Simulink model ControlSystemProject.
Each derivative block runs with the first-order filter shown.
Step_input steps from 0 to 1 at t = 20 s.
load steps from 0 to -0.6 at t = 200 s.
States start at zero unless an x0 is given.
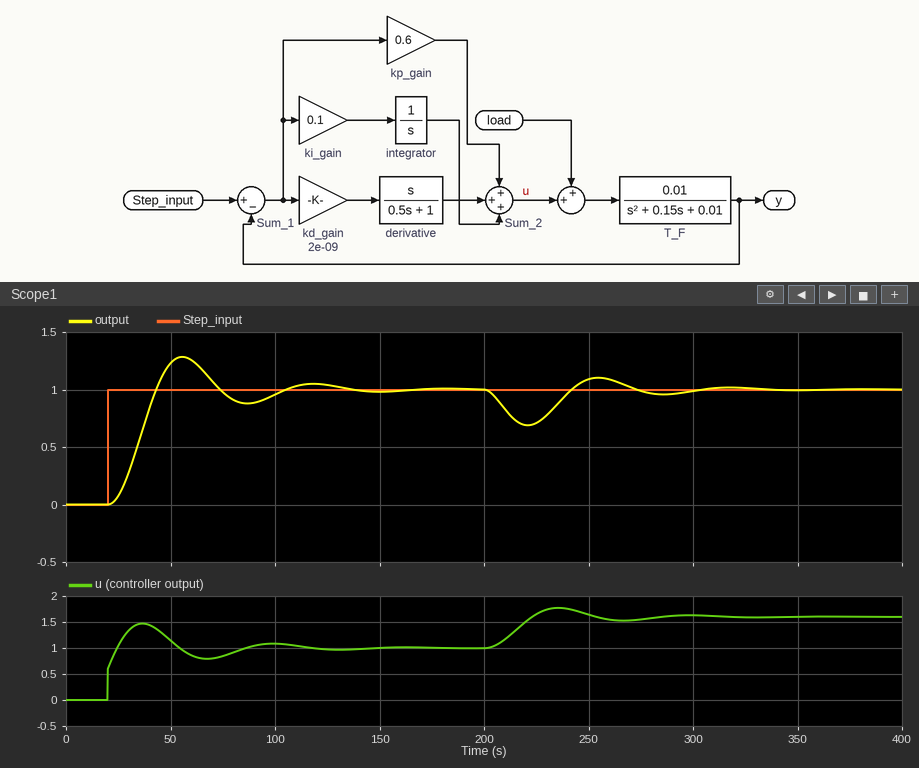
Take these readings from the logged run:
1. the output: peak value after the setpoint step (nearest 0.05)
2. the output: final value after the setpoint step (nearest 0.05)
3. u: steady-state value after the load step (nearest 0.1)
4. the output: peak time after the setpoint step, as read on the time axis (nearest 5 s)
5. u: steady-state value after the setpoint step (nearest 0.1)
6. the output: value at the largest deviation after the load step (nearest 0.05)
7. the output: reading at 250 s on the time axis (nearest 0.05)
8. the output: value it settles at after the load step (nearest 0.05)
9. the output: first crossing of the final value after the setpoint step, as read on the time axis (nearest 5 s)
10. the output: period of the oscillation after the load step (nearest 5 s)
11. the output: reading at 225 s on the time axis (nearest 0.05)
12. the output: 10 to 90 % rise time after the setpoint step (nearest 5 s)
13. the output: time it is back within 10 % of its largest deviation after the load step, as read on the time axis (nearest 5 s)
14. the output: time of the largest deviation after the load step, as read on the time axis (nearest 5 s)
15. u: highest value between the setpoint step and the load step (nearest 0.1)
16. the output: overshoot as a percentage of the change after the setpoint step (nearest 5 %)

1.30
1.00
1.6
55 s
1.0
0.70
1.10
1.00
45 s
65 s
0.70
15 s
295 s
220 s
1.5
30 %
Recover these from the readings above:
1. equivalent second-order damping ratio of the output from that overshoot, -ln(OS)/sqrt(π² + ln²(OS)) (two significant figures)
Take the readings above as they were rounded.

0.36
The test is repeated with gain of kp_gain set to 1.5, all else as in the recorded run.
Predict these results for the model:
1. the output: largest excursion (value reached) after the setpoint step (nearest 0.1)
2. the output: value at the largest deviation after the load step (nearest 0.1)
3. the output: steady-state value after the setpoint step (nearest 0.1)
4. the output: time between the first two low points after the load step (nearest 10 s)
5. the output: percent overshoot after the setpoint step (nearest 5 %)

1.1
0.8
1.0
50 s
15 %
